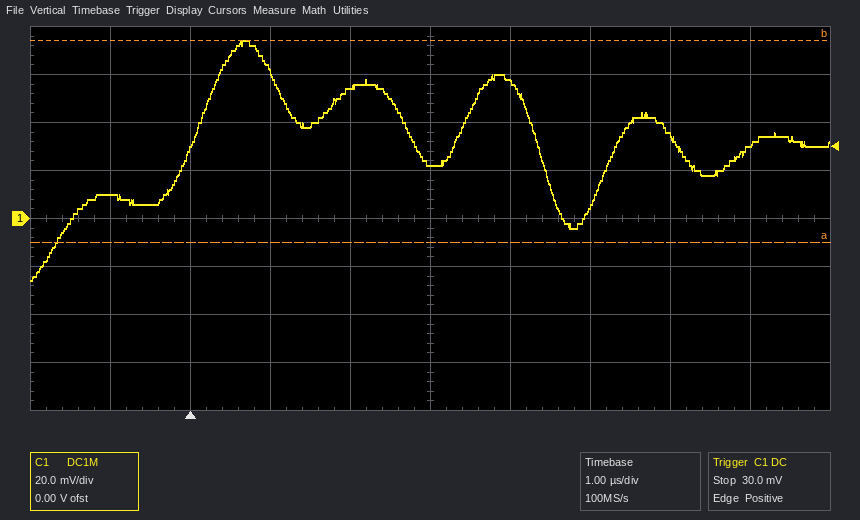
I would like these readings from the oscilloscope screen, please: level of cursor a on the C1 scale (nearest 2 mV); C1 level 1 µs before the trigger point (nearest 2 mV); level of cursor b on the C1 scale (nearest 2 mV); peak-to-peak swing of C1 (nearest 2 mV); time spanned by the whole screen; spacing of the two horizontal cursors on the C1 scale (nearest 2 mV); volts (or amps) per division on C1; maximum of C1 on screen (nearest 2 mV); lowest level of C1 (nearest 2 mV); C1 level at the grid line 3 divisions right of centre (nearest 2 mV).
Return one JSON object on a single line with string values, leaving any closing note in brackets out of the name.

{"level of cursor a on the C1 scale": "-10 mV", "C1 level 1 µs before the trigger point": "10 mV", "level of cursor b on the C1 scale": "74 mV", "peak-to-peak swing of C1": "100 mV", "time spanned by the whole screen": "10 µs", "spacing of the two horizontal cursors on the C1 scale": "84 mV", "volts (or amps) per division on C1": "20 mV", "maximum of C1 on screen": "74 mV", "lowest level of C1": "-26 mV", "C1 level at the grid line 3 divisions right of centre": "34 mV"}
